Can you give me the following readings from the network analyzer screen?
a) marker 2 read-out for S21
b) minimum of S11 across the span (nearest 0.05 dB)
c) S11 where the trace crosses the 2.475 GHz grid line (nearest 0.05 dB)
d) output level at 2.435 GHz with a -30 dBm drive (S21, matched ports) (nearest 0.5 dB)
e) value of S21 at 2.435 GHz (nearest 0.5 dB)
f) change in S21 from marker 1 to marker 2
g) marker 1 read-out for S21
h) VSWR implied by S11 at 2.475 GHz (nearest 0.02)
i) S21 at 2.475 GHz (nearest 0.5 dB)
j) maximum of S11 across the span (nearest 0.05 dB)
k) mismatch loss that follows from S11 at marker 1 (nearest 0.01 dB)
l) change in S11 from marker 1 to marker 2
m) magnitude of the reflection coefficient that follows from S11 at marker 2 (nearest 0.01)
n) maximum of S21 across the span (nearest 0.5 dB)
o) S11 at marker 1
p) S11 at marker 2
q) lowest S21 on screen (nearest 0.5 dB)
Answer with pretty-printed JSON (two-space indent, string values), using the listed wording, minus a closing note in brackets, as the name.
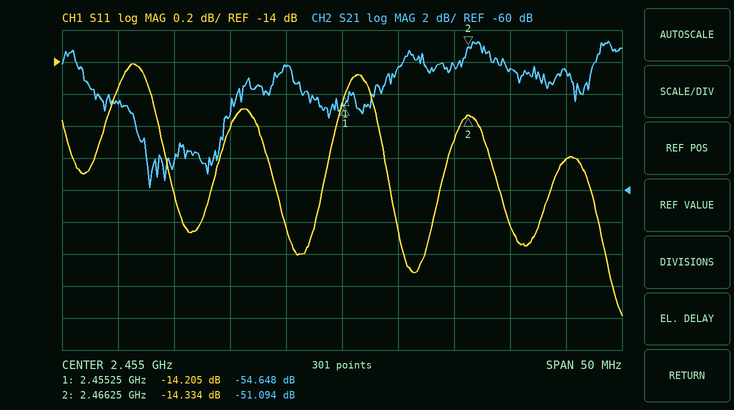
{
  "marker 2 read-out for S21": "-51.094 dB",
  "minimum of S11 across the span": "-15.60 dB",
  "S11 where the trace crosses the 2.475 GHz grid line": "-14.60 dB",
  "output level at 2.435 GHz with a -30 dBm drive (S21, matched ports)": "-84.5 dBm",
  "value of S21 at 2.435 GHz": "-54.5 dB",
  "change in S21 from marker 1 to marker 2": "3.554 dB",
  "marker 1 read-out for S21": "-54.648 dB",
  "VSWR implied by S11 at 2.475 GHz": "1.46",
  "S21 at 2.475 GHz": "-52.5 dB",
  "maximum of S11 across the span": "-14.00 dB",
  "mismatch loss that follows from S11 at marker 1": "0.17 dB",
  "change in S11 from marker 1 to marker 2": "-0.129 dB",
  "magnitude of the reflection coefficient that follows from S11 at marker 2": "0.19",
  "maximum of S21 across the span": "-50.5 dB",
  "S11 at marker 1": "-14.205 dB",
  "S11 at marker 2": "-14.334 dB",
  "lowest S21 on screen": "-60.0 dB"
}
